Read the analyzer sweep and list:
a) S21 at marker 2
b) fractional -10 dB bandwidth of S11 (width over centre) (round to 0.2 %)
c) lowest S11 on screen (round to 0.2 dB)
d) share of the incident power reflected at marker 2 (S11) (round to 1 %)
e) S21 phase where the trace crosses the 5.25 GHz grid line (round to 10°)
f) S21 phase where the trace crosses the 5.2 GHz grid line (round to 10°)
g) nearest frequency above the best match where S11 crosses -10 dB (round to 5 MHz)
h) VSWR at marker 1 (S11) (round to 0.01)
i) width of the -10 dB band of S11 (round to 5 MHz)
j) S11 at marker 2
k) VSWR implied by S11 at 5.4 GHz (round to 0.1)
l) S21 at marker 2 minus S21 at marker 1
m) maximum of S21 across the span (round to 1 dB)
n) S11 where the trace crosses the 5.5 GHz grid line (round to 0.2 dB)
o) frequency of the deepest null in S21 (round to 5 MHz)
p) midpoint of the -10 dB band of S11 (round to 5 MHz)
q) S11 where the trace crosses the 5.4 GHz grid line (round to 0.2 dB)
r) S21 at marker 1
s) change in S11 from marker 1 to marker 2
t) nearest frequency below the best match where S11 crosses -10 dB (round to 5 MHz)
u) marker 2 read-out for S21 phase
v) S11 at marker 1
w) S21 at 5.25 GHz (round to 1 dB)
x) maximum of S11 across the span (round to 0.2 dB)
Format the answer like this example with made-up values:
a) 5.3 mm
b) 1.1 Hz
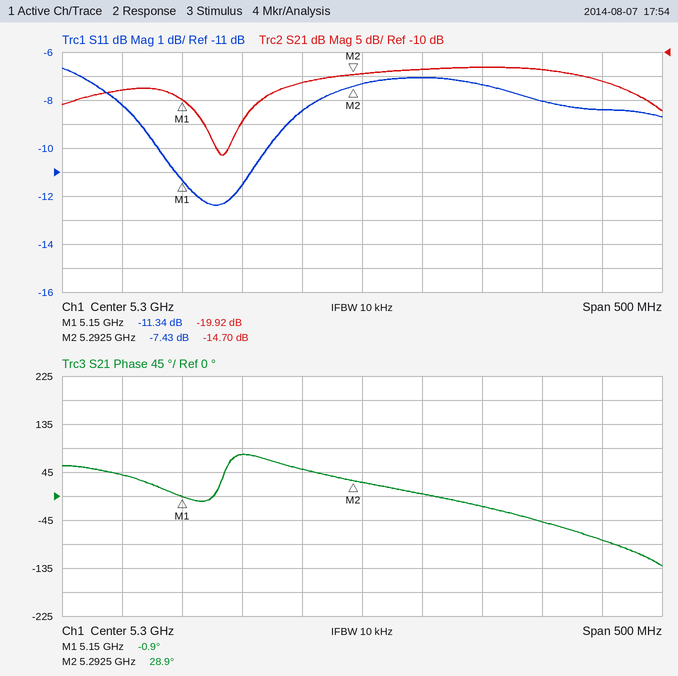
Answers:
a) -14.70 dB
b) 1.8 %
c) -12.4 dB
d) 18 %
e) 50°
f) 80°
g) 5.220 GHz
h) 1.74
i) 90 MHz
j) -7.43 dB
k) 2.5
l) 5.22 dB
m) -13 dB
n) -8.4 dB
o) 5.185 GHz
p) 5.175 GHz
q) -7.4 dB
r) -19.92 dB
s) 3.91 dB
t) 5.130 GHz
u) 28.9°
v) -11.34 dB
w) -16 dB
x) -6.6 dB
